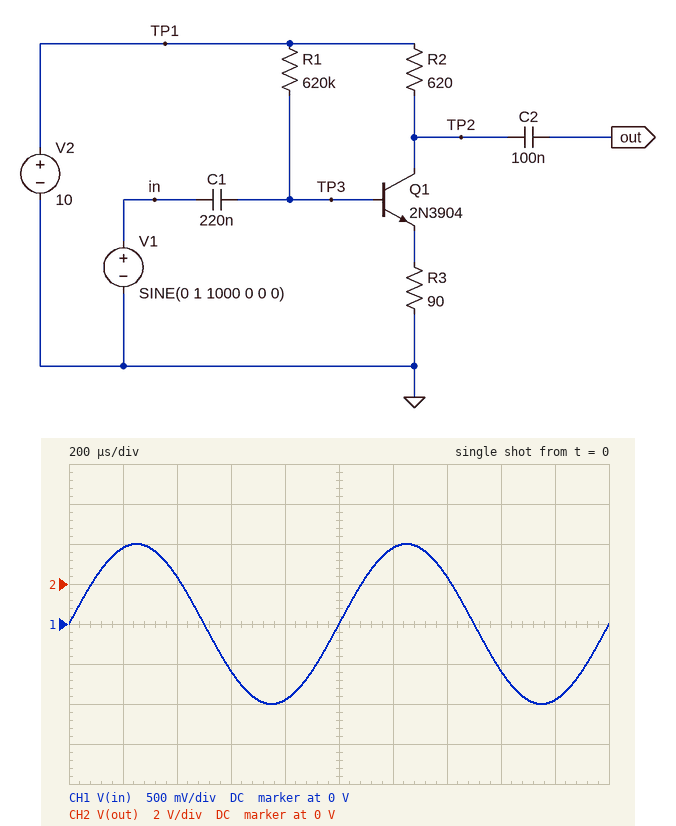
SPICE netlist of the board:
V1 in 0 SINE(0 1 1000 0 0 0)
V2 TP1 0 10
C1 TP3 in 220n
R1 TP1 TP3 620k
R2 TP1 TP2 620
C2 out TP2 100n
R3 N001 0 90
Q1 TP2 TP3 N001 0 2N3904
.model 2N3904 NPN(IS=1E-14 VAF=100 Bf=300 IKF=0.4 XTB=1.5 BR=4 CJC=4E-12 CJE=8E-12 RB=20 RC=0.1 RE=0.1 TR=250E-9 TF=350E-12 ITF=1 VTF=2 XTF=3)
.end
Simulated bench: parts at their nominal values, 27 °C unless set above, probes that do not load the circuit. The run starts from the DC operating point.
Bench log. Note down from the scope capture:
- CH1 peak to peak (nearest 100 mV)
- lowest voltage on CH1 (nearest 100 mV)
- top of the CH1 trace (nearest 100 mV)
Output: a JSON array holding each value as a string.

["2.0 V", "-1.0 V", "1.0 V"]
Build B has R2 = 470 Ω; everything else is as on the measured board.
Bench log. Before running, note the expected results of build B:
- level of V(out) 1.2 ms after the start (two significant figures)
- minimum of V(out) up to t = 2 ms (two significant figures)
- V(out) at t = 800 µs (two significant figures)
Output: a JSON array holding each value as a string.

["8.2 V", "8.0 V", "10 V"]
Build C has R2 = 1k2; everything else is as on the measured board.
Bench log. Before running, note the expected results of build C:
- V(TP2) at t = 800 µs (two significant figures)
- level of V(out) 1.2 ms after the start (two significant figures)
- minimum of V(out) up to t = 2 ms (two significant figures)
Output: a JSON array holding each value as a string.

["10 V", "5.5 V", "4.9 V"]
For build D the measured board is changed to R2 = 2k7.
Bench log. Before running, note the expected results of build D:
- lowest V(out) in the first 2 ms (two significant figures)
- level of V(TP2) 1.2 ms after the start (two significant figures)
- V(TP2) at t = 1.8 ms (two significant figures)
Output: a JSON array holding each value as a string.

["390 mV", "400 mV", "10 V"]
